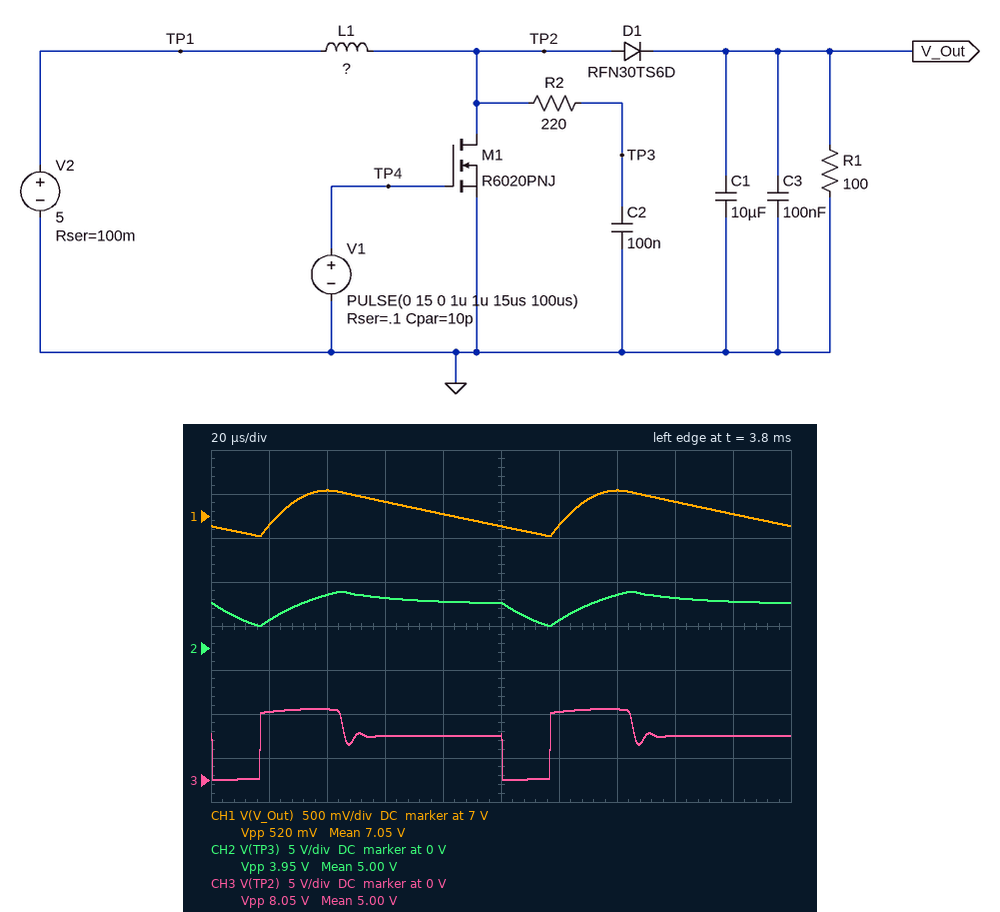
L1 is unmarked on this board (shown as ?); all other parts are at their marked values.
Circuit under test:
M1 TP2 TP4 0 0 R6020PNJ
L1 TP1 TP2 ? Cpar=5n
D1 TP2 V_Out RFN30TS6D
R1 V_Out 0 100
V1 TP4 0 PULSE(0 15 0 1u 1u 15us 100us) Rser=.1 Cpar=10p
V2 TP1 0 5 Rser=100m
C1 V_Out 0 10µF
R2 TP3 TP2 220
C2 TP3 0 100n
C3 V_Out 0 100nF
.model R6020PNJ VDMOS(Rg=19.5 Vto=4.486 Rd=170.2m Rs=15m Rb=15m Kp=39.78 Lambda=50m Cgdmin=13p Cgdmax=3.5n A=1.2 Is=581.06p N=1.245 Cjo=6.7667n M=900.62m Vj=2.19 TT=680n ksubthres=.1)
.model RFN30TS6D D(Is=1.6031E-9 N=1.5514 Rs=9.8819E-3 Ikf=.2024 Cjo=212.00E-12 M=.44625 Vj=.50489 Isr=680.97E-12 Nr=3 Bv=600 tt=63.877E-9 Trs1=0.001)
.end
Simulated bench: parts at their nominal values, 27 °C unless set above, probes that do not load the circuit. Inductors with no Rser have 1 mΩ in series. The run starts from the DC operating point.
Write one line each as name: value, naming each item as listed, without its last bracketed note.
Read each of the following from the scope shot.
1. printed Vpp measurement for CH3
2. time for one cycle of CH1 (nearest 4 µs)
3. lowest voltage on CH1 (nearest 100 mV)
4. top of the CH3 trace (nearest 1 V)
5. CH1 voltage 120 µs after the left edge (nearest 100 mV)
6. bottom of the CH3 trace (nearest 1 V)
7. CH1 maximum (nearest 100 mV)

printed Vpp measurement for CH3: 8.05 V
time for one cycle of CH1: 100 µs
lowest voltage on CH1: 6.8 V
top of the CH3 trace: 8 V
CH1 voltage 120 µs after the left edge: 6.9 V
bottom of the CH3 trace: 0 V
CH1 maximum: 7.3 V
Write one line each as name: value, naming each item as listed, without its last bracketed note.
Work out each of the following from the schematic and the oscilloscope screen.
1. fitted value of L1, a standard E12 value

fitted value of L1, a standard E12 value: 150 µH
